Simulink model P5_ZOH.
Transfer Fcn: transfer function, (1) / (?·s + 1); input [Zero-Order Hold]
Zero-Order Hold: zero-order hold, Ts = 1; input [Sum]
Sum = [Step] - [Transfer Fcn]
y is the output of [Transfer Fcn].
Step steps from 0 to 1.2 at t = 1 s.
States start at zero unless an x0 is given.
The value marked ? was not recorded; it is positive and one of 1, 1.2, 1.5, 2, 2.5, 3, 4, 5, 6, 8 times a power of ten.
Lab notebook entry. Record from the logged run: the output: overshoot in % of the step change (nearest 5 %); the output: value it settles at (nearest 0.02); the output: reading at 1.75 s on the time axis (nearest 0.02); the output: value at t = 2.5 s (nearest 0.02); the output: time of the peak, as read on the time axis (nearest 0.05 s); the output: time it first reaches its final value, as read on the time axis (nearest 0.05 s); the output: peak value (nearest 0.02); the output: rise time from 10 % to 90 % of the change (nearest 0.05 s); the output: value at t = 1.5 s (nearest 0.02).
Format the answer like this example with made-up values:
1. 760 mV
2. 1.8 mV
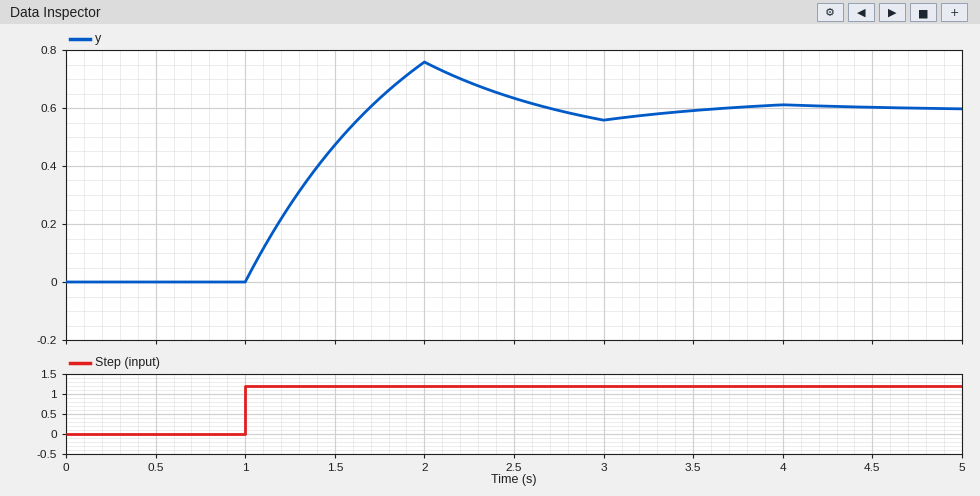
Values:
1. 25 %
2. 0.60
3. 0.64
4. 0.64
5. 2.00 s
6. 1.70 s
7. 0.76
8. 0.55 s
9. 0.48
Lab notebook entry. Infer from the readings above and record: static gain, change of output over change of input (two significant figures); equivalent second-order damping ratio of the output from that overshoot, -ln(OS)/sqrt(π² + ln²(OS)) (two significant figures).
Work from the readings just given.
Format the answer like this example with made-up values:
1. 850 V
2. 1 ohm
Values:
1. 0.50
2. 0.40
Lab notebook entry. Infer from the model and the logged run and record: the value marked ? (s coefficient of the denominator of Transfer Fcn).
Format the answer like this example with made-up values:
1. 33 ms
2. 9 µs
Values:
1. 1
